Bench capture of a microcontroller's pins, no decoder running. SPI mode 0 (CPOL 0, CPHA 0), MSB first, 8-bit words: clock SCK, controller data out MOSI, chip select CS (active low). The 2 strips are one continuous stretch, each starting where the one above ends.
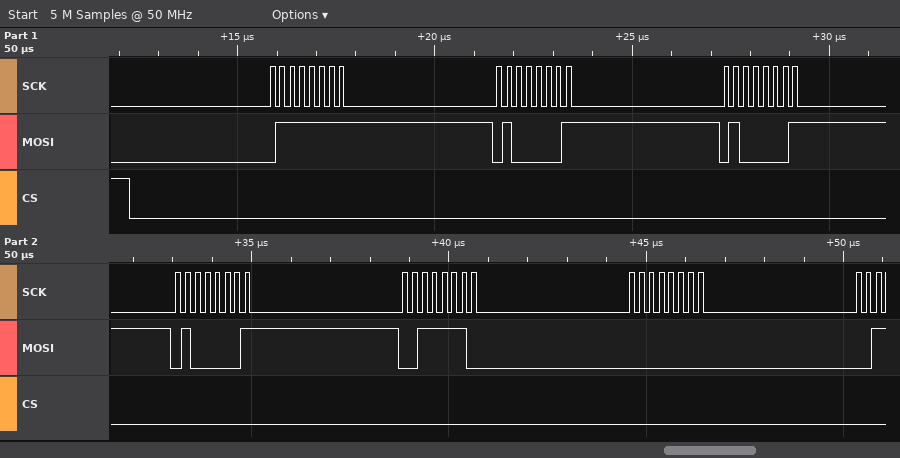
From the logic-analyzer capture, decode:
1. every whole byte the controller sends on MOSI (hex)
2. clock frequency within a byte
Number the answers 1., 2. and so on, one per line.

1. 7F 41 41 41 3E 00
2. 4 MHz
